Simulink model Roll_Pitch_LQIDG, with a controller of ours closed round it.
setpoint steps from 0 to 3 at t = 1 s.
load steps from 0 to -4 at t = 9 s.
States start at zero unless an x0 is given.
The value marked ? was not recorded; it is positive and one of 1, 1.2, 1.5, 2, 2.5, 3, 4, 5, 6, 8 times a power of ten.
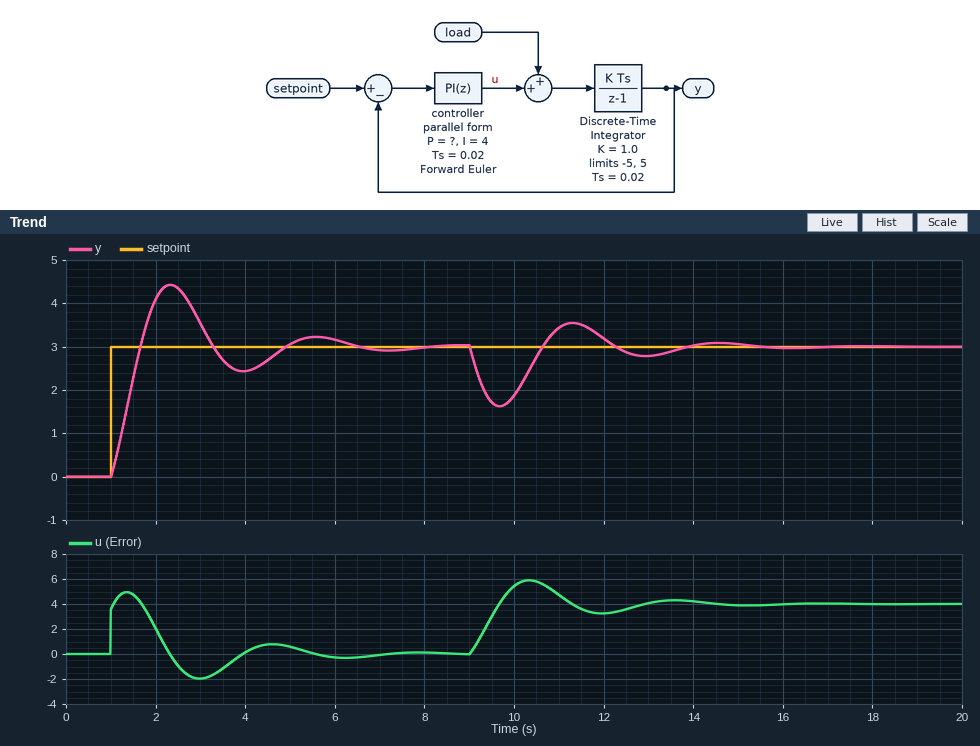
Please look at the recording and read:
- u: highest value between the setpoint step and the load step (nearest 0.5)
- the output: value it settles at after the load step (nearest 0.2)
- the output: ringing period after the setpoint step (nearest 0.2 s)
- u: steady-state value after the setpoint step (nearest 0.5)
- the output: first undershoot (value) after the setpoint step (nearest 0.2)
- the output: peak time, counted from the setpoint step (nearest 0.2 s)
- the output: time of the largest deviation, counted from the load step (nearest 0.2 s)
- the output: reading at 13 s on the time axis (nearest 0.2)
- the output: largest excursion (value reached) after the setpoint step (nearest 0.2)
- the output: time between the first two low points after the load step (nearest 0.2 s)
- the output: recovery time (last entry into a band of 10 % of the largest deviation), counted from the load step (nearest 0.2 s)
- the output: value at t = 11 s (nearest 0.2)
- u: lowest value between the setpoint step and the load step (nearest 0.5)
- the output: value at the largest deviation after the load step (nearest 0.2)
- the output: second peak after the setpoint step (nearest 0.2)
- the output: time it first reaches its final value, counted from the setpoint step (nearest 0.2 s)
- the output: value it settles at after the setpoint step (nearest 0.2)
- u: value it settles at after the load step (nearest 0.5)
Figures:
5.0
3.0
3.2 s
0.0
2.4
1.4 s
0.6 s
2.8
4.4
3.2 s
4.4 s
3.4
-2.0
1.6
3.2
0.6 s
3.0
4.0
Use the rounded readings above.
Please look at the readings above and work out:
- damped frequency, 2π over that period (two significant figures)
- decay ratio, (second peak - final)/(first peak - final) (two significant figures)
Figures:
2.0 rad/s
0.14
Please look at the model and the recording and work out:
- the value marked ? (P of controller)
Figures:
1.2
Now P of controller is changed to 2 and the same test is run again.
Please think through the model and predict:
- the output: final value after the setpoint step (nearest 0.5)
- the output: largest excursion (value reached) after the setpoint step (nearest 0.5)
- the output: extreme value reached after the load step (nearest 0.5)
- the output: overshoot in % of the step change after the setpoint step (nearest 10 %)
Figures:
3.0
4.0
2.0
30 %
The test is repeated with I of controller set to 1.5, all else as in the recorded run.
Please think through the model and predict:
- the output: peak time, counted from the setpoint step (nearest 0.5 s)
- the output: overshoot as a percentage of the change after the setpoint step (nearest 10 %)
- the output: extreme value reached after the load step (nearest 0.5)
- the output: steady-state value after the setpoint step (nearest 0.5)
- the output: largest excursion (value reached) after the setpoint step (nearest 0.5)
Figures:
2.0 s
30 %
1.0
3.0
4.0
